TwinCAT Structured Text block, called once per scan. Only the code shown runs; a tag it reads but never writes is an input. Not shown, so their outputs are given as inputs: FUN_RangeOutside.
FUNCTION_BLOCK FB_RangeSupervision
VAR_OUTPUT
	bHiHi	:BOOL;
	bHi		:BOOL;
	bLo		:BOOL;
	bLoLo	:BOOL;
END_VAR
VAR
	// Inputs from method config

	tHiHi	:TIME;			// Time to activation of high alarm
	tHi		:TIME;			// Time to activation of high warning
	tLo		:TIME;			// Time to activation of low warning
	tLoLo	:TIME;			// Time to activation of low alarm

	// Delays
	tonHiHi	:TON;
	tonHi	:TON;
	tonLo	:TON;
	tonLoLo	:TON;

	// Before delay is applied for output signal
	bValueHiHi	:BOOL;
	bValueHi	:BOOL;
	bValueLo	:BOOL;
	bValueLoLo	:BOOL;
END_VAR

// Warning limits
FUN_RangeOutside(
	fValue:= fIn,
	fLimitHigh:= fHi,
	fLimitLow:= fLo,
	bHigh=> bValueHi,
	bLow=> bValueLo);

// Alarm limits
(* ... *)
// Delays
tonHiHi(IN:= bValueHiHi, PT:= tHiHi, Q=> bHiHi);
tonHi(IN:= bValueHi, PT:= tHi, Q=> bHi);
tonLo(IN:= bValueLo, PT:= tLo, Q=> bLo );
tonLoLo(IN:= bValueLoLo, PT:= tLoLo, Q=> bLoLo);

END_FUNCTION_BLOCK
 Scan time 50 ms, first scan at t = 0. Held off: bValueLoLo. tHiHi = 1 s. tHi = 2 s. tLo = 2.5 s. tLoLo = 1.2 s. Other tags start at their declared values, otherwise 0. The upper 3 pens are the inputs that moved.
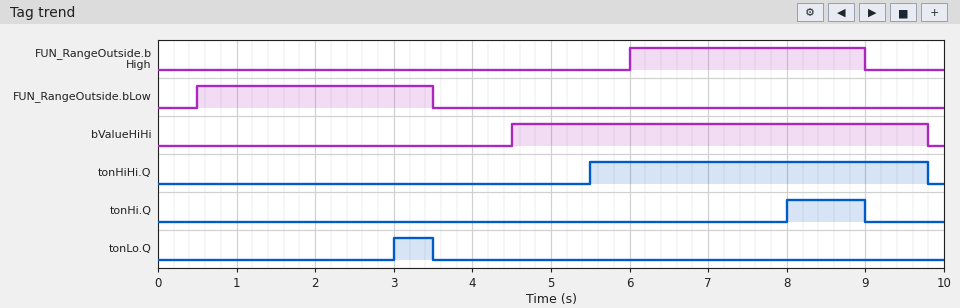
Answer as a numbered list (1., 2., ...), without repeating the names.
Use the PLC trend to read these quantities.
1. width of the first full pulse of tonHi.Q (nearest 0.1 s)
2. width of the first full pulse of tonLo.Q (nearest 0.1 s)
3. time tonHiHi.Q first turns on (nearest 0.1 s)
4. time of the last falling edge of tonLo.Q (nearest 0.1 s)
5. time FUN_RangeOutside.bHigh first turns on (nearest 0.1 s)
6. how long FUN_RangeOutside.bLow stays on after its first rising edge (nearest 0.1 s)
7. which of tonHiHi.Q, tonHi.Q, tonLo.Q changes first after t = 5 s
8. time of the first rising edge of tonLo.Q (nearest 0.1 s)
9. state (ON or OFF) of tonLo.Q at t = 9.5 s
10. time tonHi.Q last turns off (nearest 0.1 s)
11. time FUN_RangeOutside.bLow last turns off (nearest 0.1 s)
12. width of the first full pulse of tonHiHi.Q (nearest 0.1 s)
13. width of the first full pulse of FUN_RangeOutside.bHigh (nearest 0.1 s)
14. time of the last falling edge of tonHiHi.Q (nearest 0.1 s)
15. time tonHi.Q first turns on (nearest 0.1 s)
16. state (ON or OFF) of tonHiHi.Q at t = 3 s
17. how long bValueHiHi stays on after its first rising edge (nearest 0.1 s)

1. 1.0 s
2. 0.5 s
3. 5.5 s
4. 3.5 s
5. 6.0 s
6. 3.0 s
7. tonHiHi.Q
8. 3.0 s
9. OFF
10. 9.0 s
11. 3.5 s
12. 4.3 s
13. 3.0 s
14. 9.8 s
15. 8.0 s
16. OFF
17. 5.3 s
